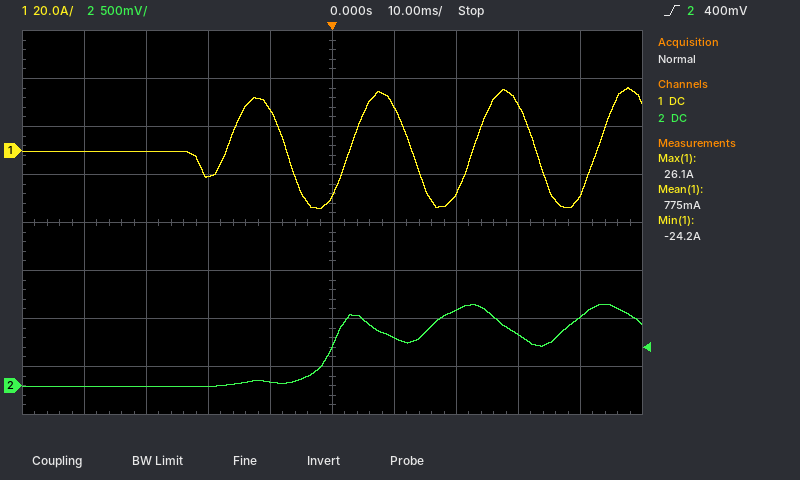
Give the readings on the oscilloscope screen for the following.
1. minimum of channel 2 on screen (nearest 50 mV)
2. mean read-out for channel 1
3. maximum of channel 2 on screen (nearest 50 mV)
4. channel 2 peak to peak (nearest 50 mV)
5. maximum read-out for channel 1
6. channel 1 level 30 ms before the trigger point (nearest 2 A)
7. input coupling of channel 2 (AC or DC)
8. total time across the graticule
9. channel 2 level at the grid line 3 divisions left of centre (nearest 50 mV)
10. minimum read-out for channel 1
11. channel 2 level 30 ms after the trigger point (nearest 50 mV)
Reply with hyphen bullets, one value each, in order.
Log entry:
- 0 mV
- 775 mA
- 850 mV
- 850 mV
- 26.1 A
- 0 A
- DC
- 100 ms
- 0 mV
- -24.2 A
- 550 mV
